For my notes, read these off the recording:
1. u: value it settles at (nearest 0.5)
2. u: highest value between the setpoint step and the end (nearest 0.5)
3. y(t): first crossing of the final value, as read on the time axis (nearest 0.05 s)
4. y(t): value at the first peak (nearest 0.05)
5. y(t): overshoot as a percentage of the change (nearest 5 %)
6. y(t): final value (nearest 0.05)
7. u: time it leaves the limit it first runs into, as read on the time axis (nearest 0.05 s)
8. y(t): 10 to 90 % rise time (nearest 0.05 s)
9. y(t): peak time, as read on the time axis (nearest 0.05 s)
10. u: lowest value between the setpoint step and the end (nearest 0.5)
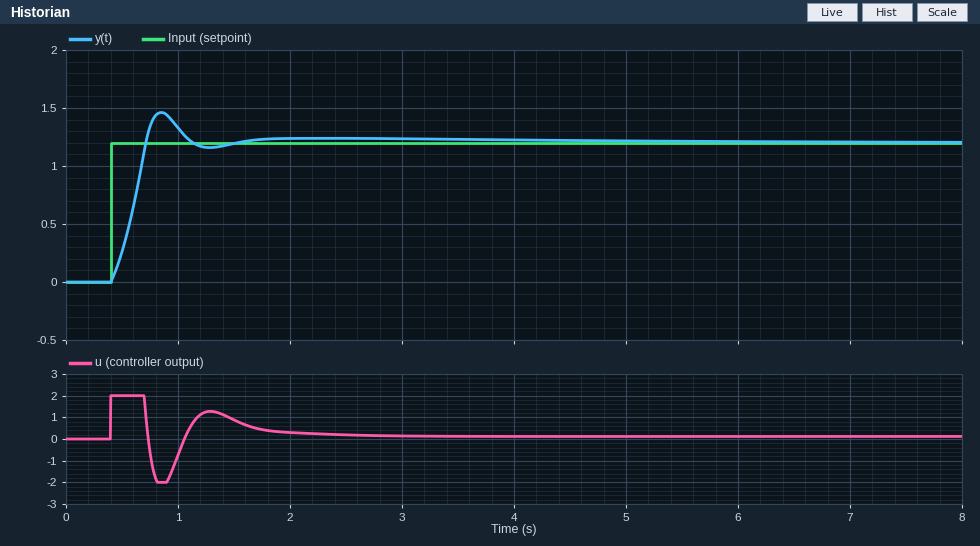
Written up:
0.0
2.0
0.70 s
1.45
20 %
1.20
0.70 s
0.25 s
0.85 s
-2.0
